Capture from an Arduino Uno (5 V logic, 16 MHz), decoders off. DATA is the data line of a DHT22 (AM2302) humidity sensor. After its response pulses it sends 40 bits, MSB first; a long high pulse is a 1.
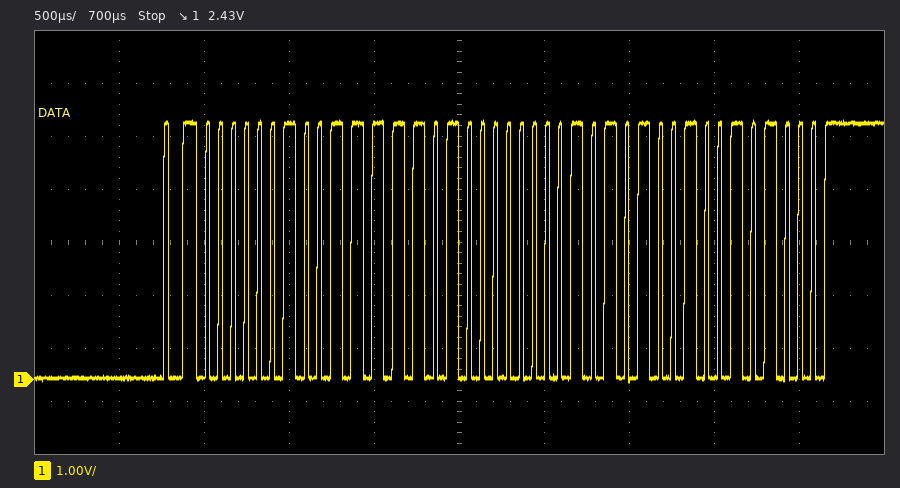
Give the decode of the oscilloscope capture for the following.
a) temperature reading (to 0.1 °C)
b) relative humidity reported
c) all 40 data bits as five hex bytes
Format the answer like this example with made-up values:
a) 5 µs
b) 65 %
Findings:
a) 16.9 °C
b) 63.7 %
c) 02 7D 00 A9 28
